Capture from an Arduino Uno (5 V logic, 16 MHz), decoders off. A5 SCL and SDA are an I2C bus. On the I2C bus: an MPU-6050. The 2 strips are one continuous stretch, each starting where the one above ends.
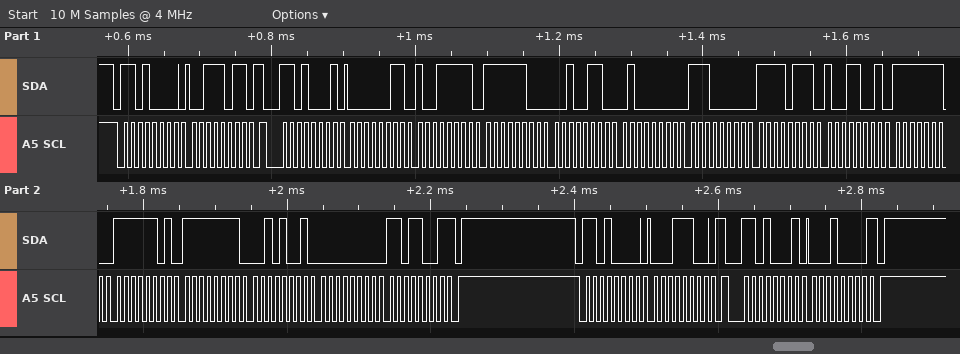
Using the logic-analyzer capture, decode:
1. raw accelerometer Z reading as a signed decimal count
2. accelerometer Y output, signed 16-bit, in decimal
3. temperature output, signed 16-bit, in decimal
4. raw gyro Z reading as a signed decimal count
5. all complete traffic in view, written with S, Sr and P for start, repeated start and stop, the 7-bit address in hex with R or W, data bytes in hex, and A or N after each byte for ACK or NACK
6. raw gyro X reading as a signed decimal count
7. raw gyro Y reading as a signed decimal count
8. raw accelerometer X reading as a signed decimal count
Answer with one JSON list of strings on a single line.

["16608", "-986", "-2151", "217", "S 68W A 3B A Sr 68R A 03 A 9F A FC A 26 A 40 A E0 A F7 A 99 A FE A FD A FF A 29 A 00 A D9 N P S 68W A 1C A Sr 68R A 10 N P", "-259", "-215", "927"]
